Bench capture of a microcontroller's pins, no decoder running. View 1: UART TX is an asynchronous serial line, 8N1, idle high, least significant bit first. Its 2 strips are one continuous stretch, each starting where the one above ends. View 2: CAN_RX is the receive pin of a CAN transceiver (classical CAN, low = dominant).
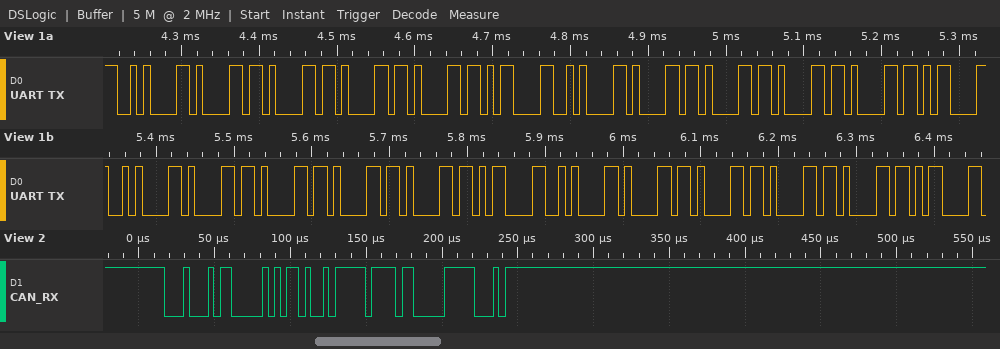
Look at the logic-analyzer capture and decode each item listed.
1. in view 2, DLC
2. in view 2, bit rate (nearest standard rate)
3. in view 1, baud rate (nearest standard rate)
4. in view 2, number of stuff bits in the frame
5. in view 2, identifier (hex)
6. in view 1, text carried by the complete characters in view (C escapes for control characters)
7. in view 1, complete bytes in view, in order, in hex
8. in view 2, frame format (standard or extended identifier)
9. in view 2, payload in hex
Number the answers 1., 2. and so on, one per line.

1. 2
2. 250 kbit/s
3. 115200 baud
4. 4
5. 0x116
6. "\naaaa\r\naaaa\r\naaaa\r\naaaa\r"
7. 0A 61 61 61 61 0D 0A 61 61 61 61 0D 0A 61 61 61 61 0D 0A 61 61 61 61 0D
8. standard
9. D2 FF
